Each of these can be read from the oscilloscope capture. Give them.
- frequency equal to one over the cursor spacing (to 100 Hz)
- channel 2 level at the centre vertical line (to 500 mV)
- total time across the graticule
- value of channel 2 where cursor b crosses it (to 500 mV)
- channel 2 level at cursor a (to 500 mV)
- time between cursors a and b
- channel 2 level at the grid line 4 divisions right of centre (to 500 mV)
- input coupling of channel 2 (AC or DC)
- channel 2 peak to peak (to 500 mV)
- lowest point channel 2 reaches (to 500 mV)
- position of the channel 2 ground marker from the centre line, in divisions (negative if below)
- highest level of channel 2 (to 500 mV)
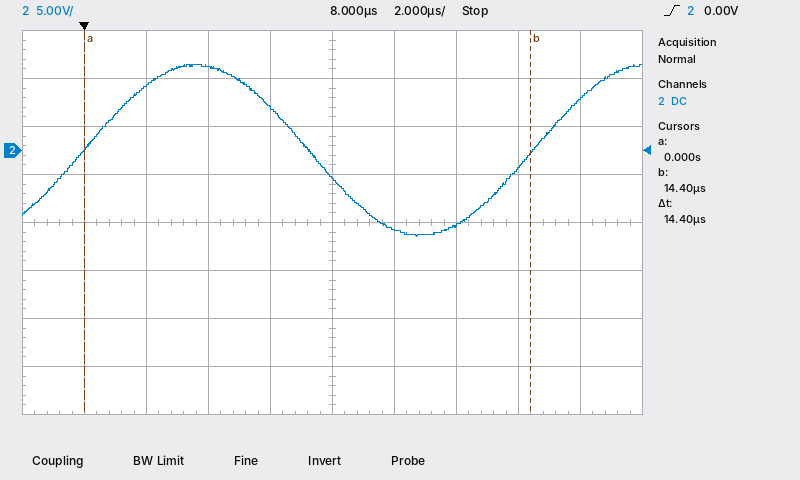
69.4 kHz
-3.0 V
20 µs
-500 mV
0.0 V
14.4 µs
5.5 V
DC
18.0 V
-9.0 V
+1.5 div
9.0 V
